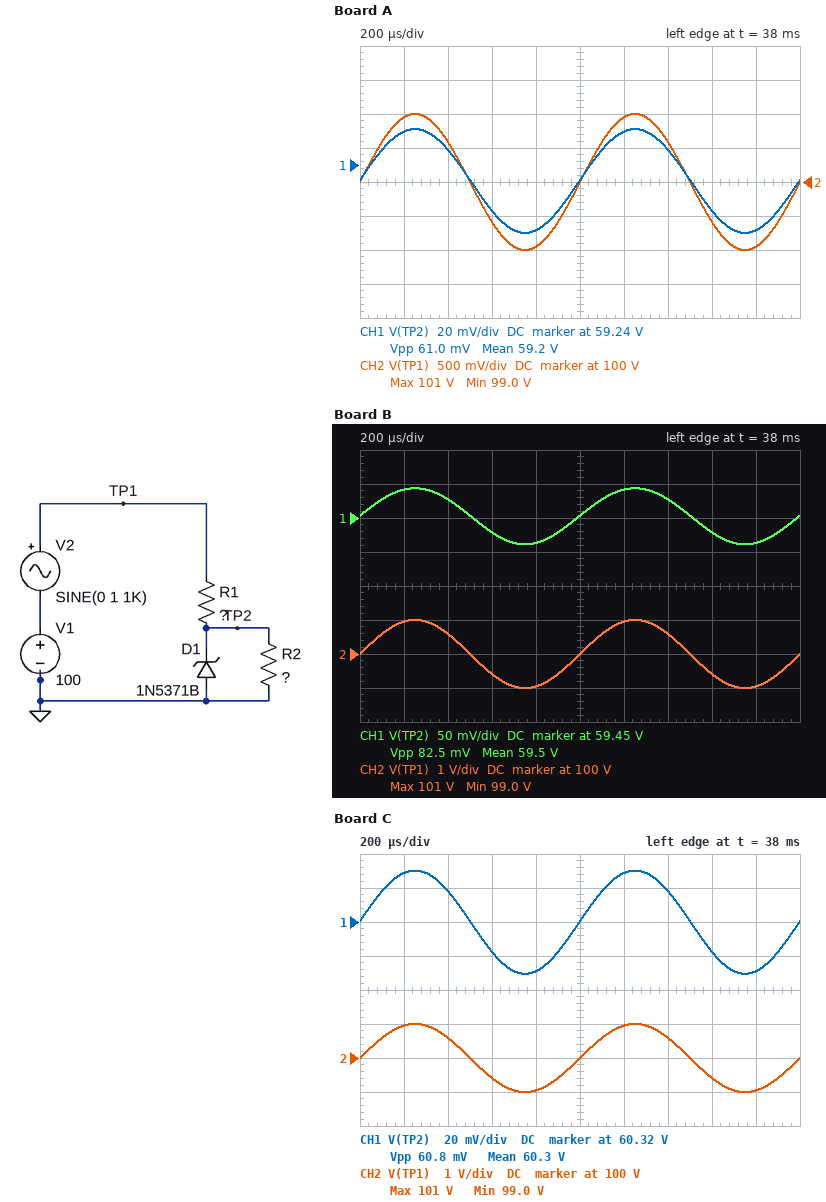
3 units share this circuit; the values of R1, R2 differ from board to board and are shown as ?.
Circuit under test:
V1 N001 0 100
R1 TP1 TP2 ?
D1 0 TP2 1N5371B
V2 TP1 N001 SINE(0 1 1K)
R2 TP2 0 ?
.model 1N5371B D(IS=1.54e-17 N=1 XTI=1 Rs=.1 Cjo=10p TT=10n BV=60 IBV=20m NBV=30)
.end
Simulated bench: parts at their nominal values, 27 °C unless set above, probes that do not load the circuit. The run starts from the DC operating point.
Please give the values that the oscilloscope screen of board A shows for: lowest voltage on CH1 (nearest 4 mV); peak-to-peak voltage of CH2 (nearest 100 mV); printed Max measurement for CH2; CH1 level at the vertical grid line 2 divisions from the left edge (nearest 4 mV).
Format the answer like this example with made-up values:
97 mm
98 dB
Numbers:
59.200 V
2.0 V
101 V
59.248 V
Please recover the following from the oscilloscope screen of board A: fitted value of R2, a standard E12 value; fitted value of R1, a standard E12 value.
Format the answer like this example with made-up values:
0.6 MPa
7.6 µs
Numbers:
12 kΩ
3.3 kΩ
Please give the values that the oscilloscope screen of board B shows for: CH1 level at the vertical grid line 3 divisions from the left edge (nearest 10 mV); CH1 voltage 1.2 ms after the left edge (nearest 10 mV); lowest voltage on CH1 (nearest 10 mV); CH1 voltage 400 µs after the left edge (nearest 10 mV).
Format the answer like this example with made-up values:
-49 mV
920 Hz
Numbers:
59.43 V
59.49 V
59.41 V
59.48 V
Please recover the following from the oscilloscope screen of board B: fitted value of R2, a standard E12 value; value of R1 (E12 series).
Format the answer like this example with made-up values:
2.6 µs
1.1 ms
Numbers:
4.7 kΩ
1.8 kΩ
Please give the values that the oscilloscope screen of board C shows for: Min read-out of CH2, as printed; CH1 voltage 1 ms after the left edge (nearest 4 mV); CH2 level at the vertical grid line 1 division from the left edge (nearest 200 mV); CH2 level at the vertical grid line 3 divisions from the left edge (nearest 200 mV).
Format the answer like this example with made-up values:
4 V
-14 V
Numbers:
99.0 V
60.320 V
101.0 V
99.4 V
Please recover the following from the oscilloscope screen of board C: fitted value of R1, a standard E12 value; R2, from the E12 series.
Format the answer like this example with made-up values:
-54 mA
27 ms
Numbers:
820 Ω
3.3 kΩ
